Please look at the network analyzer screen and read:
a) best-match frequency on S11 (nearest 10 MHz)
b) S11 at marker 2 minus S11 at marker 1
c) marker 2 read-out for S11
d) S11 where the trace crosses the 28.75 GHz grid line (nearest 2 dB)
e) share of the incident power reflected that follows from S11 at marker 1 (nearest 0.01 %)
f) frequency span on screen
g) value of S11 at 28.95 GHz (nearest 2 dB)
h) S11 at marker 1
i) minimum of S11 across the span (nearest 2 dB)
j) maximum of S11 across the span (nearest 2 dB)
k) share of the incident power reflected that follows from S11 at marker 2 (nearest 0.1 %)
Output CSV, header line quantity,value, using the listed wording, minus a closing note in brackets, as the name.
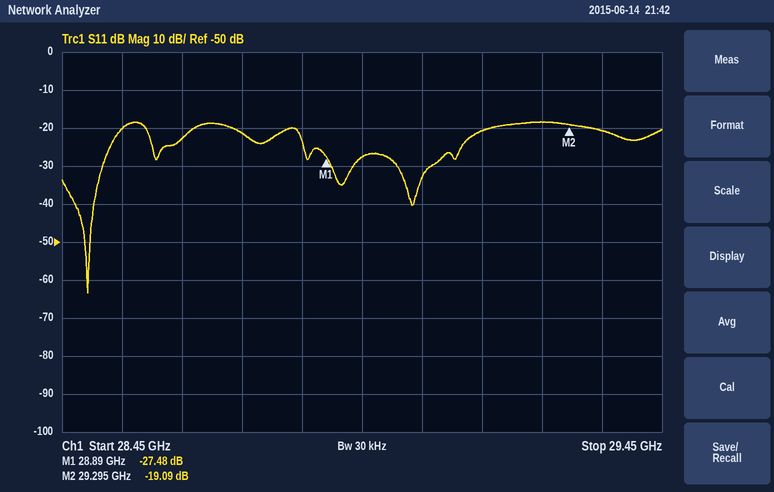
quantity,value
best-match frequency on S11,28.49 GHz
S11 at marker 2 minus S11 at marker 1,8.39 dB
marker 2 read-out for S11,-19.09 dB
S11 where the trace crosses the 28.75 GHz grid line,-22 dB
share of the incident power reflected that follows from S11 at marker 1,0.18 %
frequency span on screen,1 GHz
value of S11 at 28.95 GHz,-28 dB
S11 at marker 1,-27.48 dB
minimum of S11 across the span,-64 dB
maximum of S11 across the span,-18 dB
share of the incident power reflected that follows from S11 at marker 2,1.2 %
